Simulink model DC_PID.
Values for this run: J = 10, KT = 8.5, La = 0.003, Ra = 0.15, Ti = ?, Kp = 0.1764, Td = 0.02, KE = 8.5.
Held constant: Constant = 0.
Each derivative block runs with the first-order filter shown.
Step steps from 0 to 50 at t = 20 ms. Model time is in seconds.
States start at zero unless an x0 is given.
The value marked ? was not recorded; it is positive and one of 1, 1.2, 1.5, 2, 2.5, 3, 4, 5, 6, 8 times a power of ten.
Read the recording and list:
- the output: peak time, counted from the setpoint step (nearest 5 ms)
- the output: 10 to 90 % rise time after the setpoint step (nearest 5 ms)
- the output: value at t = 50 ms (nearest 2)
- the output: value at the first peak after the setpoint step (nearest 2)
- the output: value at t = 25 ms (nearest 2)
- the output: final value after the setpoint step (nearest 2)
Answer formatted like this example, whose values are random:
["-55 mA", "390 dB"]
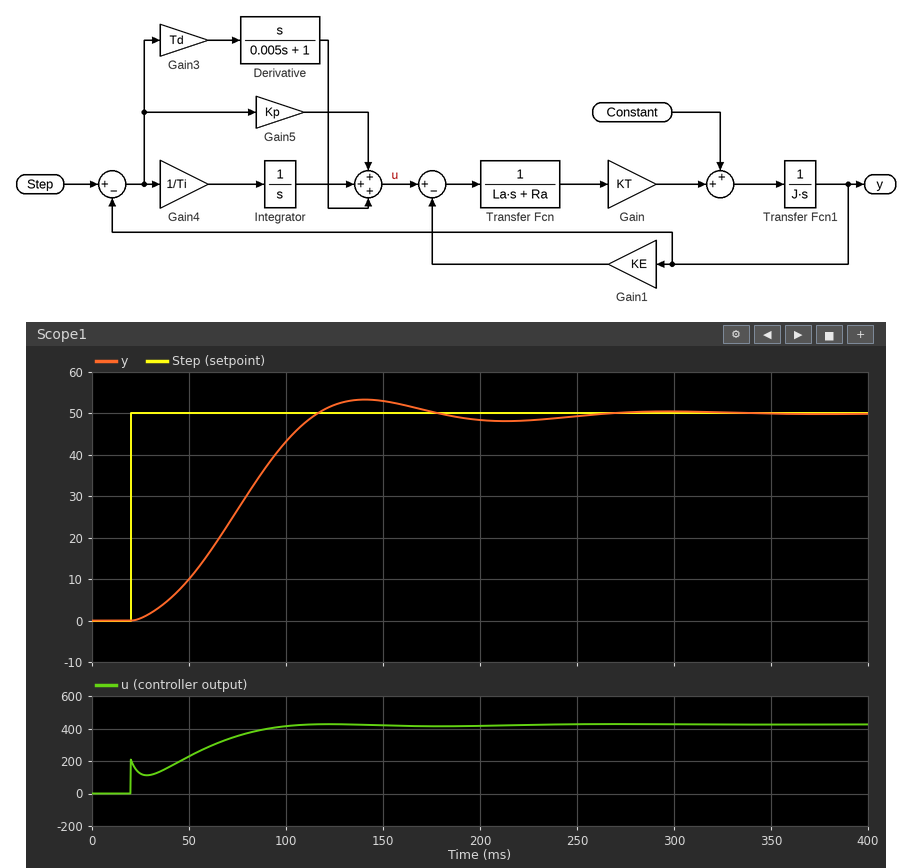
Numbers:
["120 ms", "65 ms", "10", "54", "0", "50"]
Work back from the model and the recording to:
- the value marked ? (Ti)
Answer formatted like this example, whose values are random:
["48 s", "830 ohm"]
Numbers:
["0.006"]
